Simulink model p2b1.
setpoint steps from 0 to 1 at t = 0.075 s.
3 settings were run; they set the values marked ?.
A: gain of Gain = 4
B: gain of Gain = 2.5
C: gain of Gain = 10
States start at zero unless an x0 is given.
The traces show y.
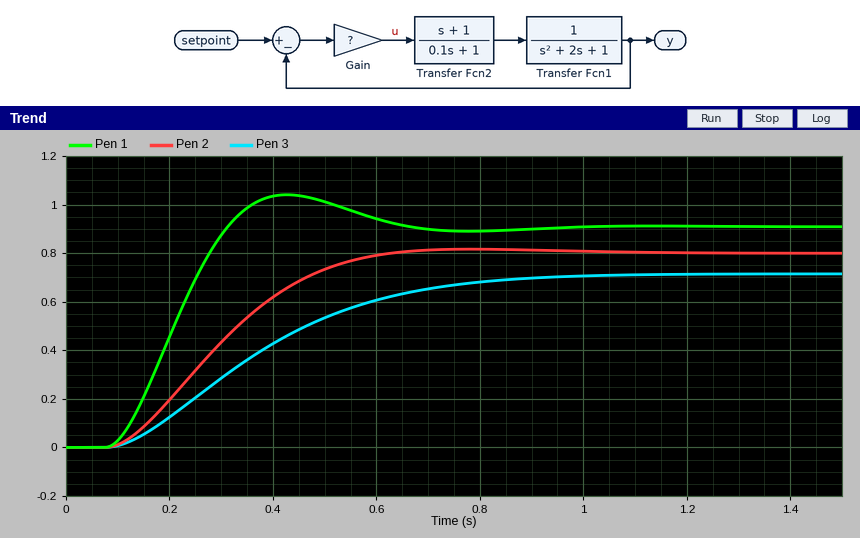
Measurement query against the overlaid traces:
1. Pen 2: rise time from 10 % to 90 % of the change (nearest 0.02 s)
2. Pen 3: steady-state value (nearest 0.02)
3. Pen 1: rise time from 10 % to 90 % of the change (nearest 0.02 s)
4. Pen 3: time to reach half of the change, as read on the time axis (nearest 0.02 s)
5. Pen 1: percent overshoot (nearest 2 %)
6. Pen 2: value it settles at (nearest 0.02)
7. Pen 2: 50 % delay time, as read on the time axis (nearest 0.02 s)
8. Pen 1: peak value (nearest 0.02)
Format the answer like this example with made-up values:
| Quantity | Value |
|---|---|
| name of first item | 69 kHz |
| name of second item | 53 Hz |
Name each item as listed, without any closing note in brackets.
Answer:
| Quantity | Value |
|---|---|
| Pen 2: rise time from 10 % to 90 % of the change | 0.34 s |
| Pen 3: steady-state value | 0.72 |
| Pen 1: rise time from 10 % to 90 % of the change | 0.16 s |
| Pen 3: time to reach half of the change, as read on the time axis | 0.34 s |
| Pen 1: percent overshoot | 14 % |
| Pen 2: value it settles at | 0.80 |
| Pen 2: 50 % delay time, as read on the time axis | 0.28 s |
| Pen 1: peak value | 1.04 |
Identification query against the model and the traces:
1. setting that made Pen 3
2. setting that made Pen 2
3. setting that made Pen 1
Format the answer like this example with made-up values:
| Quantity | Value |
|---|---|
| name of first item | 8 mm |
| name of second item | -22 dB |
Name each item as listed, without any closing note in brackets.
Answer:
| Quantity | Value |
|---|---|
| setting that made Pen 3 | B |
| setting that made Pen 2 | A |
| setting that made Pen 1 | C |
